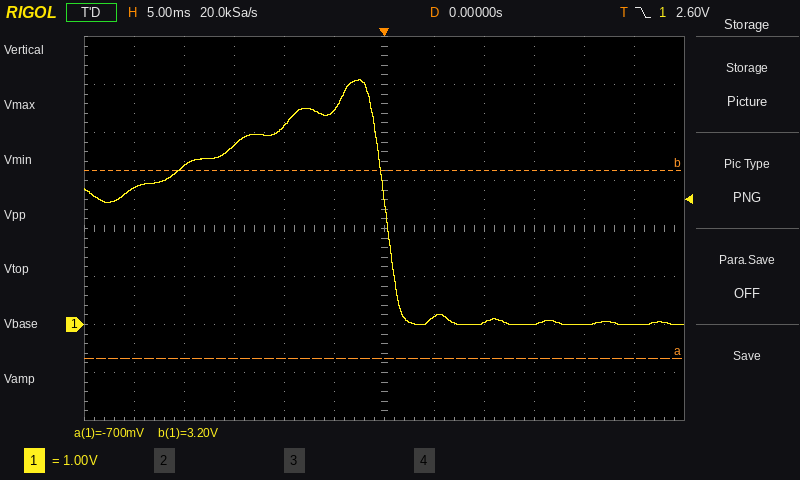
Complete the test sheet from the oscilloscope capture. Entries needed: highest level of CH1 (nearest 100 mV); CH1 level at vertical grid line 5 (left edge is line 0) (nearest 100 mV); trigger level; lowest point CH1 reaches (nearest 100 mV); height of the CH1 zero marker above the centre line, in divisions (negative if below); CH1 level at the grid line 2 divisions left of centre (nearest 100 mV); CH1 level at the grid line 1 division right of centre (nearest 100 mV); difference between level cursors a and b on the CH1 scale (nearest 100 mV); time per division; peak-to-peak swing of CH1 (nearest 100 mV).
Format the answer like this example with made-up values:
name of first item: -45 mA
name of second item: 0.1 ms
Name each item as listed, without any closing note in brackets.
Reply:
highest level of CH1: 5.1 V
CH1 level at vertical grid line 5 (left edge is line 0): 4.5 V
trigger level: 2.60 V
lowest point CH1 reaches: 0.0 V
height of the CH1 zero marker above the centre line, in divisions: -2.0 div
CH1 level at the grid line 2 divisions left of centre: 4.1 V
CH1 level at the grid line 1 division right of centre: 200 mV
difference between level cursors a and b on the CH1 scale: 3.9 V
time per division: 5 ms
peak-to-peak swing of CH1: 5.1 V
